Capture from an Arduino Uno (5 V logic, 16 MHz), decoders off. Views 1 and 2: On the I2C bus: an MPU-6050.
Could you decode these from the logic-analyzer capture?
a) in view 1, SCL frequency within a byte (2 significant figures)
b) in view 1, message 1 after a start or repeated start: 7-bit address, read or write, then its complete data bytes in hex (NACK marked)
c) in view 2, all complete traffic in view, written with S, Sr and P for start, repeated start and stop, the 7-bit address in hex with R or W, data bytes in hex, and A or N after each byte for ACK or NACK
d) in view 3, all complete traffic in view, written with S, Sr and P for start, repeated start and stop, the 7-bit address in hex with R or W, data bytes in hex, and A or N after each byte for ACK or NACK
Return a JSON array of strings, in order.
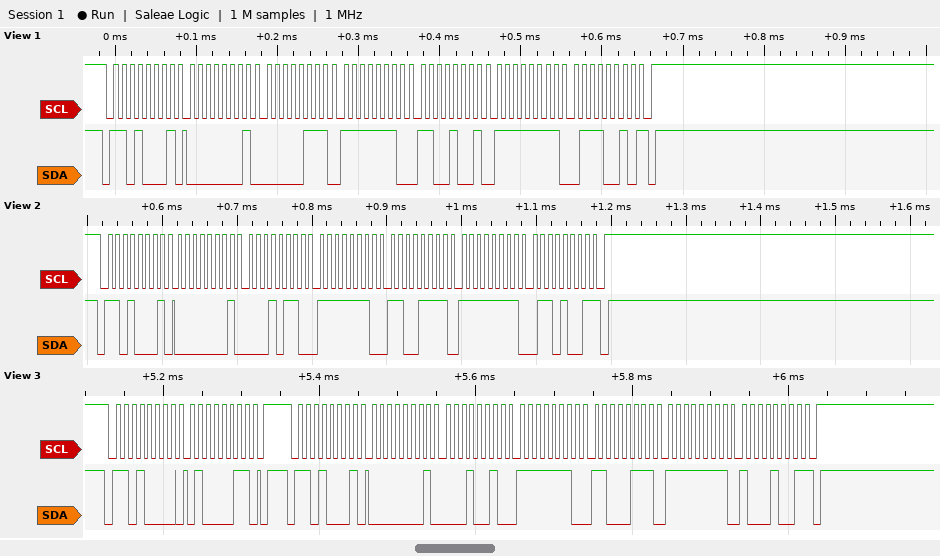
["100 kHz", "0x68 read: 01 07 FE C9 FF 72 NACK", "S 68R A 01 A 16 A FE A CF A FF A 69 N P", "S 68W A 43 A P S 68R A 01 A 12 A FE A C7 A FF A 89 N P"]
